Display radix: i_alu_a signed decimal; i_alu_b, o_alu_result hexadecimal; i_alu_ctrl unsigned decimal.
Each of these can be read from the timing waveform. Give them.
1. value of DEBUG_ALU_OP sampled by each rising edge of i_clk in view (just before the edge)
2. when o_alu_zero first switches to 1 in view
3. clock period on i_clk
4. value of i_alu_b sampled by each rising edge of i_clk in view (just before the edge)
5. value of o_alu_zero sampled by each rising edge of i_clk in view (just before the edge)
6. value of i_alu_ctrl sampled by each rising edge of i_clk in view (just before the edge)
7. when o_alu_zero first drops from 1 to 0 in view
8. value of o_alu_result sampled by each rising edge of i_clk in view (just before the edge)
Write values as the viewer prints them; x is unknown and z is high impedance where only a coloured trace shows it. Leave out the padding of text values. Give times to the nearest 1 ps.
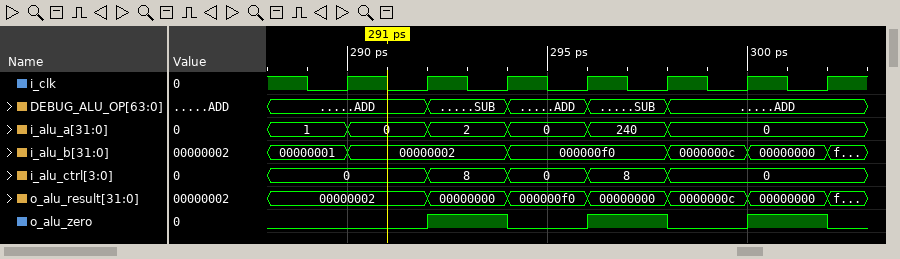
ADD, ADD, SUB, ADD, SUB, ADD, ADD
292 ps
2 ps
00000001, 00000002, 00000002, 000000f0, 000000f0, 0000000c, 00000000
0 0 1 0 1 0 1
0, 0, 8, 0, 8, 0, 0
294 ps
00000002, 00000002, 00000000, 000000f0, 00000000, 0000000c, 00000000
